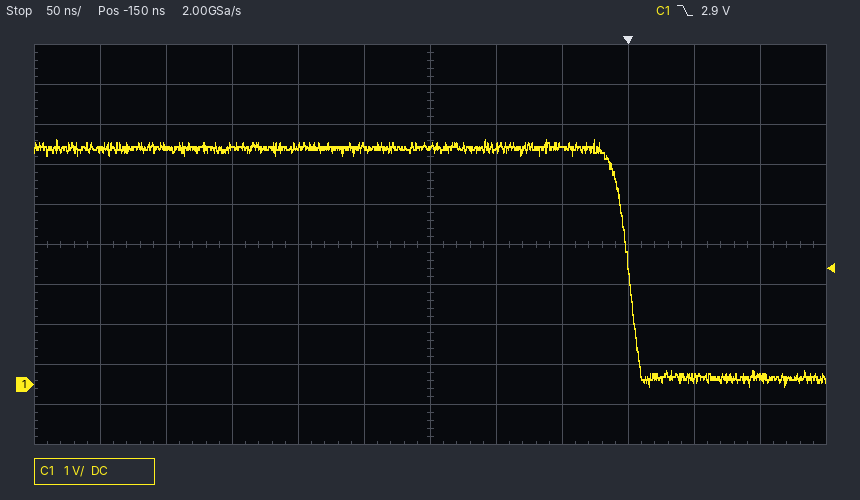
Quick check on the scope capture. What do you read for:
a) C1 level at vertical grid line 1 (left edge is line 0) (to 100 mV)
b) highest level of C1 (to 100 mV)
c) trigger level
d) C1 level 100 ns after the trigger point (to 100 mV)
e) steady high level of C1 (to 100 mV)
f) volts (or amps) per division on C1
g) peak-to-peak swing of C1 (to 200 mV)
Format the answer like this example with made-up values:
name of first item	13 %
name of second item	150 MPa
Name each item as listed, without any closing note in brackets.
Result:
C1 level at vertical grid line 1 (left edge is line 0)	5.9 V
highest level of C1	6.1 V
trigger level	2.9 V
C1 level 100 ns after the trigger point	200 mV
steady high level of C1	5.9 V
volts (or amps) per division on C1	1 V
peak-to-peak swing of C1	6.2 V
